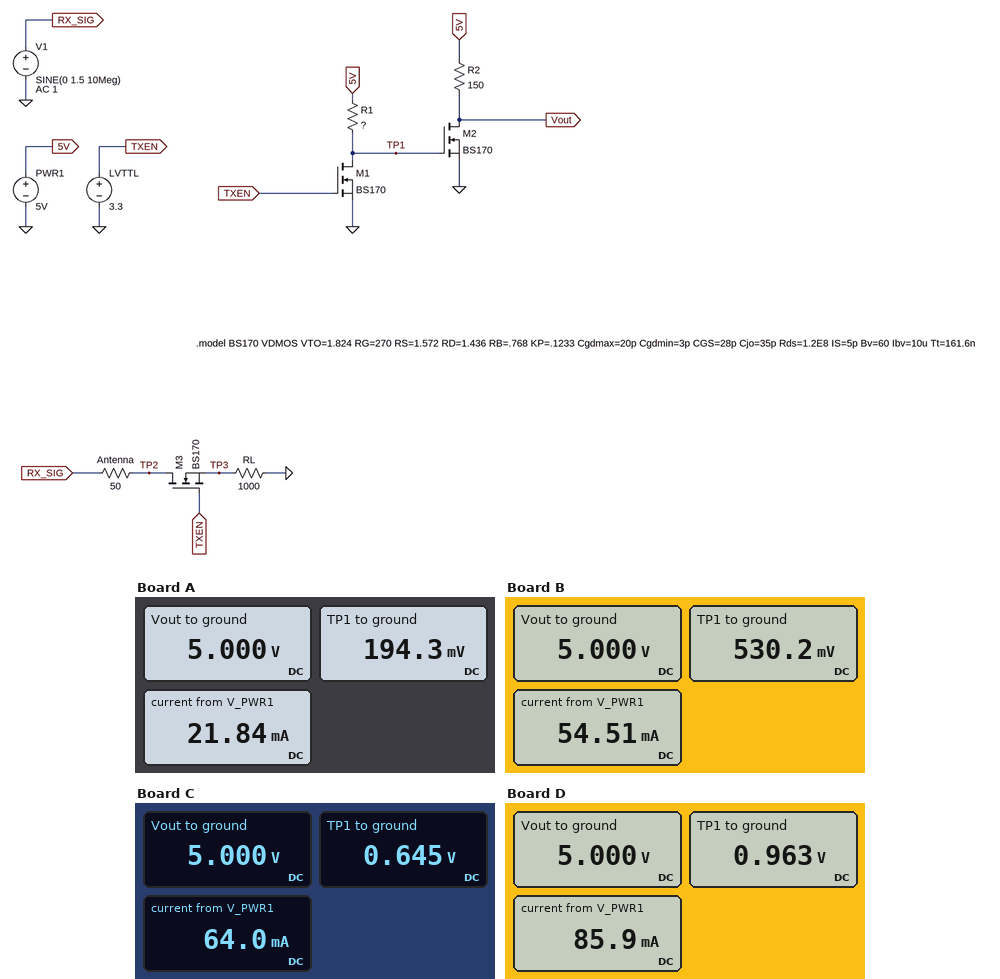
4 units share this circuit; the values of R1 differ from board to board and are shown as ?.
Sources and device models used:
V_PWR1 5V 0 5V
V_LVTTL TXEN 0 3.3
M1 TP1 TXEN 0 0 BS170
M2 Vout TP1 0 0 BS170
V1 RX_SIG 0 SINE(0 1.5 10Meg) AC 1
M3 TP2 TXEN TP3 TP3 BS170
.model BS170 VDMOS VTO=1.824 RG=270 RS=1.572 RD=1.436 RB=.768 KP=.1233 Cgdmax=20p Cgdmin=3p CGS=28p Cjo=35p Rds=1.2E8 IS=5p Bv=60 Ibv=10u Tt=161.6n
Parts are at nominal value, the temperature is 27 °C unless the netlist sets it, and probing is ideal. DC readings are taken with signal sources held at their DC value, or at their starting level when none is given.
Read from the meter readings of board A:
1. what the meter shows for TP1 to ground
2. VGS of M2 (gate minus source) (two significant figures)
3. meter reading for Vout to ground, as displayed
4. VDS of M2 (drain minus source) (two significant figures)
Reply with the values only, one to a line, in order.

194.3 mV
190 mV
5.000 V
5.0 V
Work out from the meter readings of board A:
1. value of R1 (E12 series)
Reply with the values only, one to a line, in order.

220 Ω
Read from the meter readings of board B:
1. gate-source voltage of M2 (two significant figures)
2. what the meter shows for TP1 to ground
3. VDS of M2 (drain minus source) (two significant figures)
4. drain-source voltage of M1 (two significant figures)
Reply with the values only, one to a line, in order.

530 mV
530.2 mV
5.0 V
530 mV
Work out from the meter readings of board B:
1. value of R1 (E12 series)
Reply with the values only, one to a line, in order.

82 Ω
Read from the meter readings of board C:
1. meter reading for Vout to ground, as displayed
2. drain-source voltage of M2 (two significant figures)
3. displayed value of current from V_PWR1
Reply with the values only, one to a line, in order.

5.000 V
5.0 V
64.0 mA
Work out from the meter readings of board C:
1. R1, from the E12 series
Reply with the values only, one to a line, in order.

68 Ω
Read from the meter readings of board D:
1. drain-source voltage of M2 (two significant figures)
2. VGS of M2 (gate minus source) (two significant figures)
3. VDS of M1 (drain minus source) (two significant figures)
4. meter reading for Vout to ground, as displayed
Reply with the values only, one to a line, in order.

5.0 V
960 mV
960 mV
5.000 V
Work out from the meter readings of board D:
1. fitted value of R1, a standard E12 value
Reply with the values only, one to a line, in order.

47 Ω
